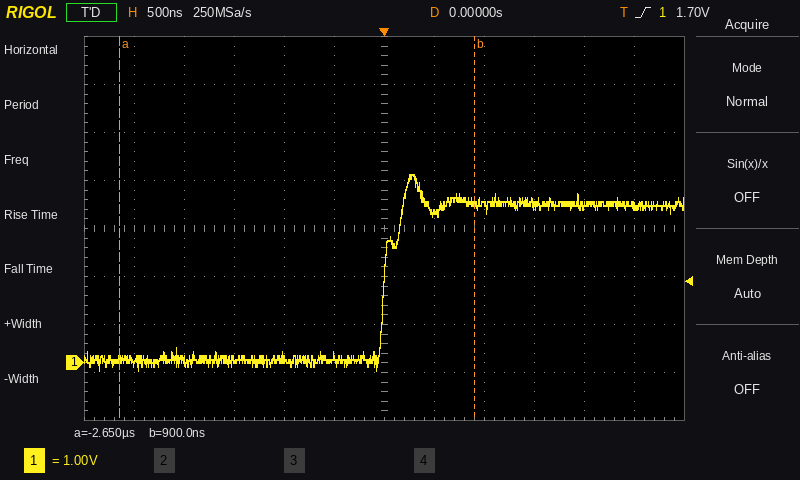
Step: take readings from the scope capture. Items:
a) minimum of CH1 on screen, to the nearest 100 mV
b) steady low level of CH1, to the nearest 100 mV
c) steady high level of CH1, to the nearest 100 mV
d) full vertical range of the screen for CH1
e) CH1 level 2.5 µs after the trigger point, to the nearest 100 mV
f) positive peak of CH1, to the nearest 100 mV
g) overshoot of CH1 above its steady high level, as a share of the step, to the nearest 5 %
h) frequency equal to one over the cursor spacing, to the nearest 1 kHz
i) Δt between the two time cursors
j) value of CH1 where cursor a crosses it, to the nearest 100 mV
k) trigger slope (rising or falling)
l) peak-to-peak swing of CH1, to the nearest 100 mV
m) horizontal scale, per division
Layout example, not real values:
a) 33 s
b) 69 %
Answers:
a) -200 mV
b) 100 mV
c) 3.3 V
d) 8 V
e) 3.3 V
f) 3.9 V
g) 20 %
h) 282 kHz
i) 3.55 µs
j) 100 mV
k) rising
l) 4.1 V
m) 500 ns
